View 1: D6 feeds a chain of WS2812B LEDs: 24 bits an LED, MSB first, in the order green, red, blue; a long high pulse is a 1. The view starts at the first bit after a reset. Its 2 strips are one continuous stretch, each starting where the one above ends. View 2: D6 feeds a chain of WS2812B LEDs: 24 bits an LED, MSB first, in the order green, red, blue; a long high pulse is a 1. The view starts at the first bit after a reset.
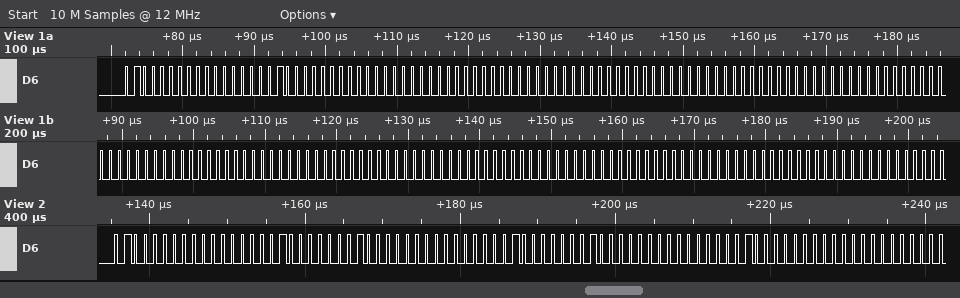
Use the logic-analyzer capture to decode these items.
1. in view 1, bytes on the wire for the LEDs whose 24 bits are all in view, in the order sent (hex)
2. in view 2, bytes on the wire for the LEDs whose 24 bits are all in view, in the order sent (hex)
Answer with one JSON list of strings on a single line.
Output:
["40 00 40 00 00 00 00 00 00 00 00 00 00 00 00 00 00 00 00 00 00", "40 00 40 40 00 40 40 00 40"]
